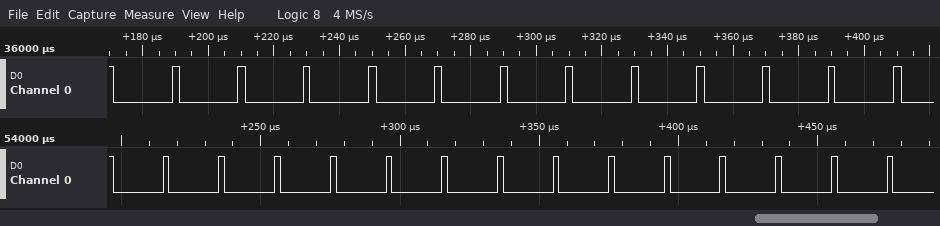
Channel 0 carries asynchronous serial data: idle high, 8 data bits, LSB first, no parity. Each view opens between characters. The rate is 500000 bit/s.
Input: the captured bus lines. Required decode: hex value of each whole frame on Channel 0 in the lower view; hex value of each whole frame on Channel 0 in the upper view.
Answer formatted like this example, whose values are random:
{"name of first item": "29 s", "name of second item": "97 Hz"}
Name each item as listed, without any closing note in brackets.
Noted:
{"hex value of each whole frame on Channel 0 in the lower view": "00, 00, 00, 00, 00, 00, 00, 00, 00, 00, 00, 00, 00, 00", "hex value of each whole frame on Channel 0 in the upper view": "00, 00, 00, 00, 00, 00, 00, 00, 00, 00, 00, 00"}
